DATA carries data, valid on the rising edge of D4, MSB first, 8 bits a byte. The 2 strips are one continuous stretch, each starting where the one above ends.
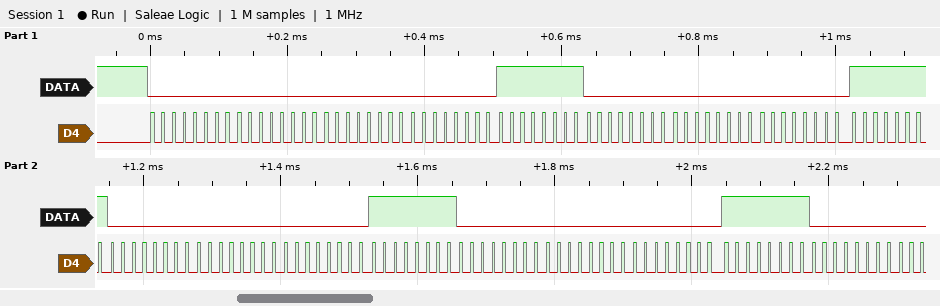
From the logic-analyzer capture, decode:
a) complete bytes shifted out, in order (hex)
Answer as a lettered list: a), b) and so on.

a) 00 00 00 00 FF 00 00 00 FF 00 00 00 FF 00 00 00 FF 00
